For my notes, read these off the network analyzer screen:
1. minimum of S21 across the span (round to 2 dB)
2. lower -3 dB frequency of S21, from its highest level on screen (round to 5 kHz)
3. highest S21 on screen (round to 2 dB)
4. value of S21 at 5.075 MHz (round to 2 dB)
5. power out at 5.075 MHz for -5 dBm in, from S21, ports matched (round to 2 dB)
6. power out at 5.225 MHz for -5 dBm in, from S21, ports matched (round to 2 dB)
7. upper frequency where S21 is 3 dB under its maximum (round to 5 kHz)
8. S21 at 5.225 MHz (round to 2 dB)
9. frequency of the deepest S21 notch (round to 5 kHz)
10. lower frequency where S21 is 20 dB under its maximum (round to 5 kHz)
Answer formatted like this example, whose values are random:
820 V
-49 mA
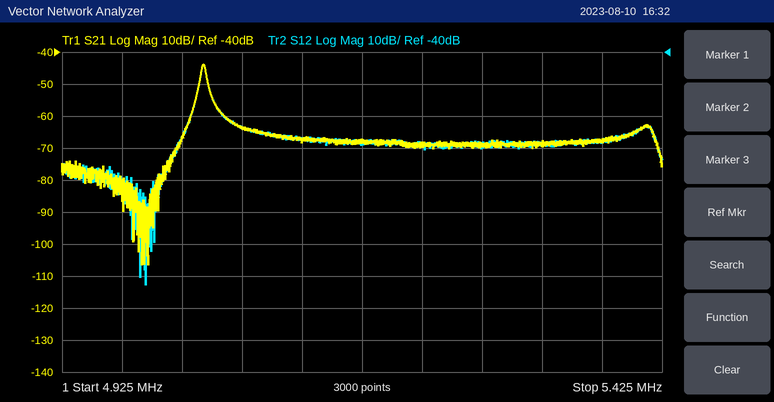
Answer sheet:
-106 dB
5.040 MHz
-44 dB
-64 dB
-68 dBm
-74 dBm
5.045 MHz
-68 dB
4.990 MHz
5.030 MHz
